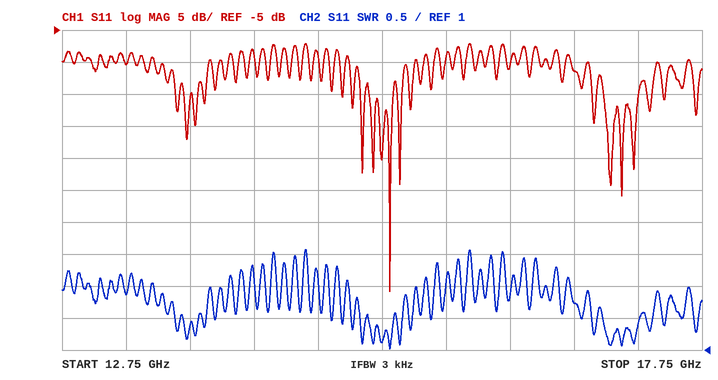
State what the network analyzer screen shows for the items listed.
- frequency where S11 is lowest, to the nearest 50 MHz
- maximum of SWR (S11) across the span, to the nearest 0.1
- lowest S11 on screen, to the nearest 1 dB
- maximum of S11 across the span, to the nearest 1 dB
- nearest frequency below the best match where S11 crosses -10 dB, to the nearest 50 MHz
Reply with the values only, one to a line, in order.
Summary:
15.30 GHz
2.6
-46 dB
-7 dB
15.00 GHz
